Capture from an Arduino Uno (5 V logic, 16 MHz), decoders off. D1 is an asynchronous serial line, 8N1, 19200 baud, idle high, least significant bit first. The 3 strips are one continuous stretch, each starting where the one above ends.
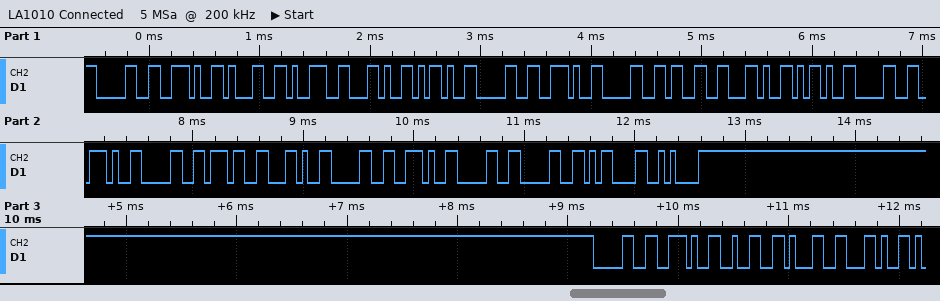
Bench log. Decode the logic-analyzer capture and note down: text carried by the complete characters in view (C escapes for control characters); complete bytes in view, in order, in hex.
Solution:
"0.19,-0.03,-0.07,0.00\r\n0.21,"
0x30 0x2E 0x31 0x39 0x2C 0x2D 0x30 0x2E 0x30 0x33 0x2C 0x2D 0x30 0x2E 0x30 0x37 0x2C 0x30 0x2E 0x30 0x30 0x0D 0x0A 0x30 0x2E 0x32 0x31 0x2C
